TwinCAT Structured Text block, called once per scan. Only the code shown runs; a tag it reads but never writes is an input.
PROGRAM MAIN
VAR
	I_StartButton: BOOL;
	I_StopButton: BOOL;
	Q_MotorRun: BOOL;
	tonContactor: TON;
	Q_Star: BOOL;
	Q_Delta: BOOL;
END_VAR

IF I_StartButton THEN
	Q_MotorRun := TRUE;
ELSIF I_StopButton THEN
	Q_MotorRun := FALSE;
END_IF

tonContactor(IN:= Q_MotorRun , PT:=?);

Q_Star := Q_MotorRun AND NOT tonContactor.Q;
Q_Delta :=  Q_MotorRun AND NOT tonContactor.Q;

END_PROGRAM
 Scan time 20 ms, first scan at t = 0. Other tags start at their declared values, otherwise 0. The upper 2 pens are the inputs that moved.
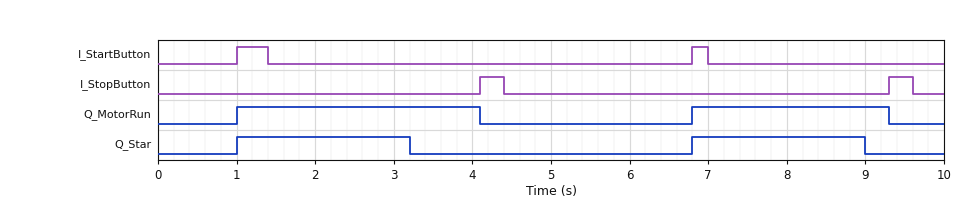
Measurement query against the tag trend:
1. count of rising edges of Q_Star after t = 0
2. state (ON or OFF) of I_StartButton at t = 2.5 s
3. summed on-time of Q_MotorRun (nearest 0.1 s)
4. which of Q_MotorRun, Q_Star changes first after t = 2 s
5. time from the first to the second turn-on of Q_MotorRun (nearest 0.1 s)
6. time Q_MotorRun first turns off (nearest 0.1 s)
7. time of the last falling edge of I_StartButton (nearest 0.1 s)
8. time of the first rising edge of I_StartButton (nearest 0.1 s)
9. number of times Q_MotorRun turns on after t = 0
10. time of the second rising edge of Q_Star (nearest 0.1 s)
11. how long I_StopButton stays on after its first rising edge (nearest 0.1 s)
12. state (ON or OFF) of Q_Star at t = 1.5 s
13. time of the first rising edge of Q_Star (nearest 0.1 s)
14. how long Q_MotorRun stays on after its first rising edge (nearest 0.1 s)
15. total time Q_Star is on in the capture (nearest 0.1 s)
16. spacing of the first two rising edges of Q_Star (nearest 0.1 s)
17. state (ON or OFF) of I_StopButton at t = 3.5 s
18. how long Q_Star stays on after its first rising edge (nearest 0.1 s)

2
OFF
5.6 s
Q_Star
5.8 s
4.1 s
7.0 s
1.0 s
2
6.8 s
0.3 s
ON
1.0 s
3.1 s
4.4 s
5.8 s
OFF
2.2 s
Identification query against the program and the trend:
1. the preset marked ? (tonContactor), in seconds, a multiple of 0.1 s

2.2 s
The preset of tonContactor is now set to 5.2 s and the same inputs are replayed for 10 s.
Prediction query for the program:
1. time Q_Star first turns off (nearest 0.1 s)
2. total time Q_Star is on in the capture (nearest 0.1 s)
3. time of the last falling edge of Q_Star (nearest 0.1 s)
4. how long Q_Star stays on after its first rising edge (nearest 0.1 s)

4.1 s
5.6 s
9.3 s
3.1 s
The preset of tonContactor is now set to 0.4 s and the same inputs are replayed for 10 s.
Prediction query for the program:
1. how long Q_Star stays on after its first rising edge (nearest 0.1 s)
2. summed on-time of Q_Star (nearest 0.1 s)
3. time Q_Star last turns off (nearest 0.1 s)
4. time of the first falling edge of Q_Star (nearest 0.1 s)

0.4 s
0.8 s
7.2 s
1.4 s
